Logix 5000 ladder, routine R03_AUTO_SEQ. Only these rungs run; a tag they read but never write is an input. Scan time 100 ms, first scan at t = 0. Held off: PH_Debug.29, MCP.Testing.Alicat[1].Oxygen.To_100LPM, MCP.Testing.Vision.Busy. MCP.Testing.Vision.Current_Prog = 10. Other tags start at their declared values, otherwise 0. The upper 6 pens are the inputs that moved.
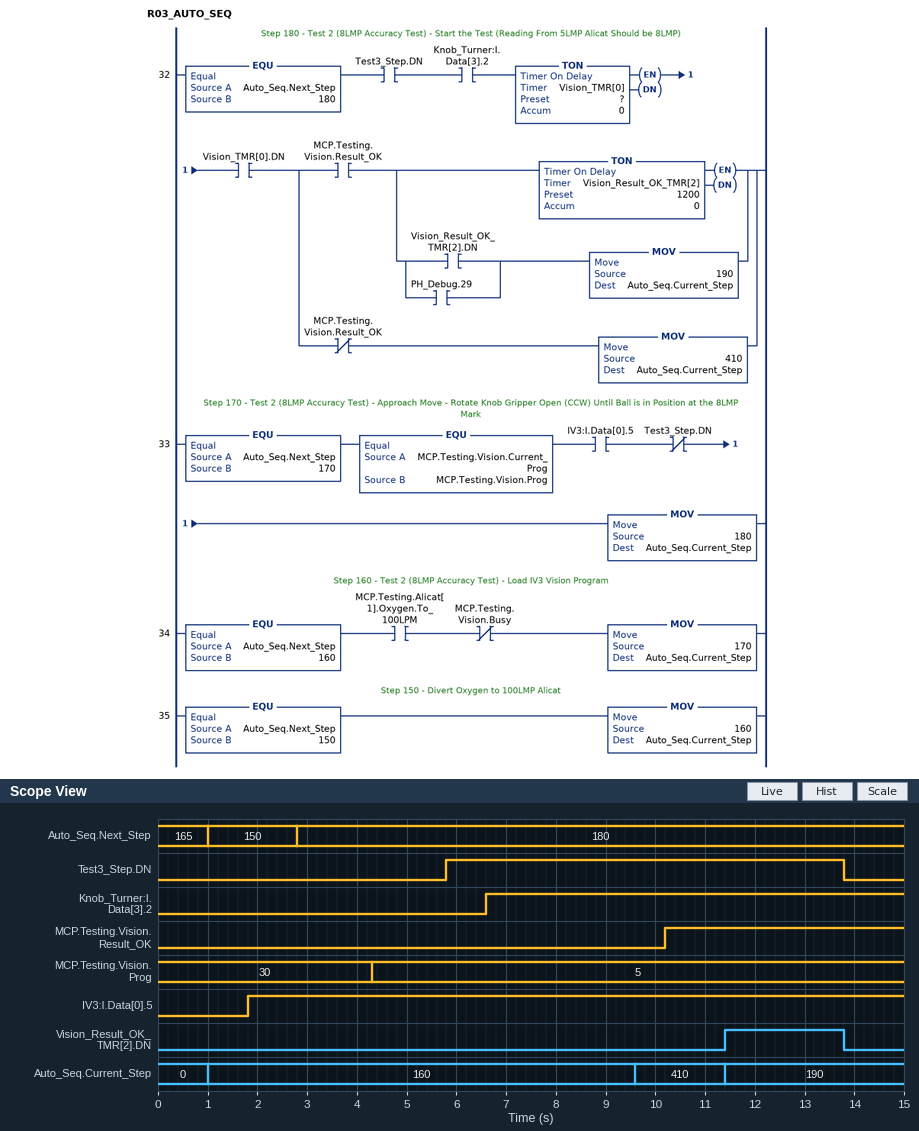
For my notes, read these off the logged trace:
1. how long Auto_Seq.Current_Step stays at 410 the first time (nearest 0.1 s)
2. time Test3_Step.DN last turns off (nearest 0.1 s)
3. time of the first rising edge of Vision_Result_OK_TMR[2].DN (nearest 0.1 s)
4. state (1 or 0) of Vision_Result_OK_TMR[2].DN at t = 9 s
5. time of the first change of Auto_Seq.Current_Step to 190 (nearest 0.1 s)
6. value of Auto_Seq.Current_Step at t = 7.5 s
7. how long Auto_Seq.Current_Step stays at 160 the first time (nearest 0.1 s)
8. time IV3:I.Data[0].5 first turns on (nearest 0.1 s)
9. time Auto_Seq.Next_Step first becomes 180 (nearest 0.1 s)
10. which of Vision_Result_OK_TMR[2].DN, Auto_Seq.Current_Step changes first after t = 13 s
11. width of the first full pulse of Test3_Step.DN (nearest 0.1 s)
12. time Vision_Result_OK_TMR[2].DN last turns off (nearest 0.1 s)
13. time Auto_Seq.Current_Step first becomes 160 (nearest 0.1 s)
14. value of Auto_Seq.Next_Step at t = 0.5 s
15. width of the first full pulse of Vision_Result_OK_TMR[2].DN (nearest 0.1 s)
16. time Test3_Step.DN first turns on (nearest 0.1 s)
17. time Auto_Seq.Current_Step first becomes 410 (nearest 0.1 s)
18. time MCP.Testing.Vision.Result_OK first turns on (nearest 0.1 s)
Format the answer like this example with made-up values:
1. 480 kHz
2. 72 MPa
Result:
1. 1.8 s
2. 13.8 s
3. 11.4 s
4. 0
5. 11.4 s
6. 160
7. 8.6 s
8. 1.8 s
9. 2.8 s
10. Vision_Result_OK_TMR[2].DN
11. 8.0 s
12. 13.8 s
13. 1.0 s
14. 165
15. 2.4 s
16. 5.8 s
17. 9.6 s
18. 10.2 s
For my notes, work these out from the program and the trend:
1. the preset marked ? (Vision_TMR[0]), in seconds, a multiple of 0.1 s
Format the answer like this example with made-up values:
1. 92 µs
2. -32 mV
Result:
1. 3.0 s
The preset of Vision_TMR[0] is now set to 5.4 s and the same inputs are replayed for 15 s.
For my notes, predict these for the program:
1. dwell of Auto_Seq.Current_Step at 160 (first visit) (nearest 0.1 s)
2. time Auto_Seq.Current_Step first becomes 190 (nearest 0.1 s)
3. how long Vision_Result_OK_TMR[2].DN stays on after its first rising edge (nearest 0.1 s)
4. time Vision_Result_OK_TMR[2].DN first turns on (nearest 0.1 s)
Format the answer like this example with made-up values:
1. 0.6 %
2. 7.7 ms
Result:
1. 12.2 s
2. 13.2 s
3. 0.6 s
4. 13.2 s
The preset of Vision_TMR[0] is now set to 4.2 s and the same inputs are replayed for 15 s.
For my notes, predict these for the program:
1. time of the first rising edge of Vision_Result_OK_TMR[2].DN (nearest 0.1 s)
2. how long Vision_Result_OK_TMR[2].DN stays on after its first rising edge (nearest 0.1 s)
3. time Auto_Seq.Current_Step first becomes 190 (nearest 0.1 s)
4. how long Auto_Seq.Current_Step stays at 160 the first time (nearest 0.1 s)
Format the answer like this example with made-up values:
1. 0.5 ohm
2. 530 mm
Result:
1. 12.0 s
2. 1.8 s
3. 12.0 s
4. 11.0 s
